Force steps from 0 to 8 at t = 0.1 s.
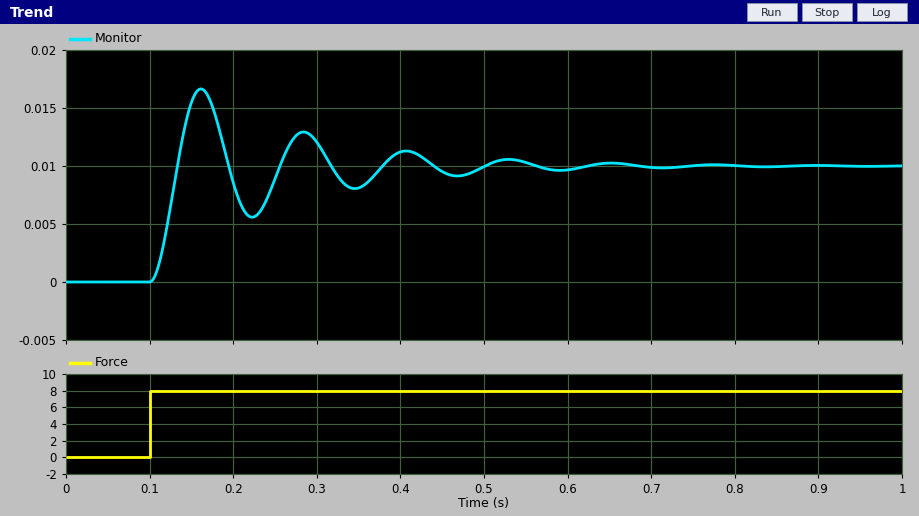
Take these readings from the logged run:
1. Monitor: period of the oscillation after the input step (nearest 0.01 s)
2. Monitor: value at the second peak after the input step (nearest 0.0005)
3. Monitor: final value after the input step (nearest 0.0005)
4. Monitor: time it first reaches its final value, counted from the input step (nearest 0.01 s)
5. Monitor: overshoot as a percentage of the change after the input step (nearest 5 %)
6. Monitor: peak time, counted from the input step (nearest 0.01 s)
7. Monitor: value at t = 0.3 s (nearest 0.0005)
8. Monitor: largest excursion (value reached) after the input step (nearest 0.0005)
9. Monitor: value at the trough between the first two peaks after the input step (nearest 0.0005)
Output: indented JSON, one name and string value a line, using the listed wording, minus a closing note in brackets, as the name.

{
  "Monitor: period of the oscillation after the input step": "0.12 s",
  "Monitor: value at the second peak after the input step": "0.0130",
  "Monitor: final value after the input step": "0.0100",
  "Monitor: time it first reaches its final value, counted from the input step": "0.03 s",
  "Monitor: overshoot as a percentage of the change after the input step": "65 %",
  "Monitor: peak time, counted from the input step": "0.06 s",
  "Monitor: value at t = 0.3 s": "0.0120",
  "Monitor: largest excursion (value reached) after the input step": "0.0165",
  "Monitor: value at the trough between the first two peaks after the input step": "0.0055"
}
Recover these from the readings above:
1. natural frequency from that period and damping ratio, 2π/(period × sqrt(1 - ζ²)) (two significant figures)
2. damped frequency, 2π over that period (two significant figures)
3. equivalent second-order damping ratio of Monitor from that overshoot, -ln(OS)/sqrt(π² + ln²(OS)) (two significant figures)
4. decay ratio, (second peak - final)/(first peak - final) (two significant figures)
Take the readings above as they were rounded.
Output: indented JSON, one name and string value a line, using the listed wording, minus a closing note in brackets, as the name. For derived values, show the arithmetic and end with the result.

{
  "natural frequency from that period and damping ratio, 2π/(period × sqrt(1 - ζ²))": "2π / (0.12 × sqrt(1 - 0.14²)) = 53 rad/s",
  "damped frequency, 2π over that period": "2π / 0.12 = 52 rad/s",
  "equivalent second-order damping ratio of Monitor from that overshoot, -ln(OS)/sqrt(π² + ln²(OS))": "ln(0.65) = -0.431; 0.431 / sqrt(9.870 + 0.186) = 0.14",
  "decay ratio, (second peak - final)/(first peak - final)": "(0.013 - 0.01) / (0.0165 - 0.01) = 0.46"
}
